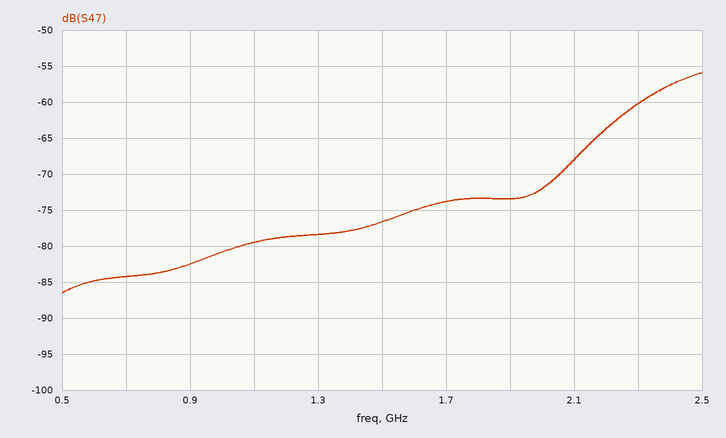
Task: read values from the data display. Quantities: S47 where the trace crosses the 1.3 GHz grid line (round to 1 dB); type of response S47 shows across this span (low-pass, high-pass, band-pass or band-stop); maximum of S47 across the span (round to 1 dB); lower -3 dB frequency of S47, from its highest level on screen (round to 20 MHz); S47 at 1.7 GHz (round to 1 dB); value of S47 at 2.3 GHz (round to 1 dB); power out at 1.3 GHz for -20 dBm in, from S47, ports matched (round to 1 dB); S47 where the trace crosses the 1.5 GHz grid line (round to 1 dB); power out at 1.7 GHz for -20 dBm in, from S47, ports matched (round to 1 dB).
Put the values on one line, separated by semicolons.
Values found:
-78 dB; high-pass; -56 dB; 2.34 GHz; -74 dB; -60 dB; -98 dBm; -77 dB; -94 dBm
